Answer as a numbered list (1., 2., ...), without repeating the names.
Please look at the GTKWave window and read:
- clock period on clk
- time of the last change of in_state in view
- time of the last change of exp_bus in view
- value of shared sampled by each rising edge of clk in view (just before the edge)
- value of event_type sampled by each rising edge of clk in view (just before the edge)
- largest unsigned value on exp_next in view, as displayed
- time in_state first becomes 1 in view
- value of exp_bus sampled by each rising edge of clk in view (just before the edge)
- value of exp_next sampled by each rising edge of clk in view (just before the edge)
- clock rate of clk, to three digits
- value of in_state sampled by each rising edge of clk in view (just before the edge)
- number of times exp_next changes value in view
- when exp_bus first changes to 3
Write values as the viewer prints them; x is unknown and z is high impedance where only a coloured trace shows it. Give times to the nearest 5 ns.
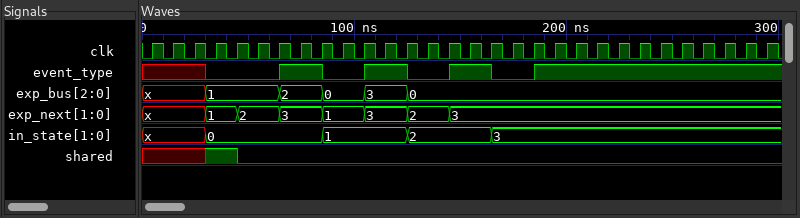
1. 10 ns
2. 165 ns
3. 125 ns
4. x x x 1 1 0 0 0 0 0 0 0 0 0 0 0 0 0 0 0 0 0 0 0 0 0 0 0 0 0
5. x x x 0 0 0 0 1 1 0 0 1 1 0 0 1 1 0 0 1 1 1 1 1 1 1 1 1 1 1
6. 3
7. 85 ns
8. x, x, x, 1, 1, 1, 1, 2, 2, 0, 0, 3, 3, 0, 0, 0, 0, 0, 0, 0, 0, 0, 0, 0, 0, 0, 0, 0, 0, 0
9. x, x, x, 1, 1, 2, 2, 3, 3, 1, 1, 3, 3, 2, 2, 3, 3, 3, 3, 3, 3, 3, 3, 3, 3, 3, 3, 3, 3, 3
10. 100 MHz
11. x, x, x, 0, 0, 0, 0, 0, 0, 1, 1, 1, 1, 2, 2, 2, 2, 3, 3, 3, 3, 3, 3, 3, 3, 3, 3, 3, 3, 3
12. 7
13. 105 ns
